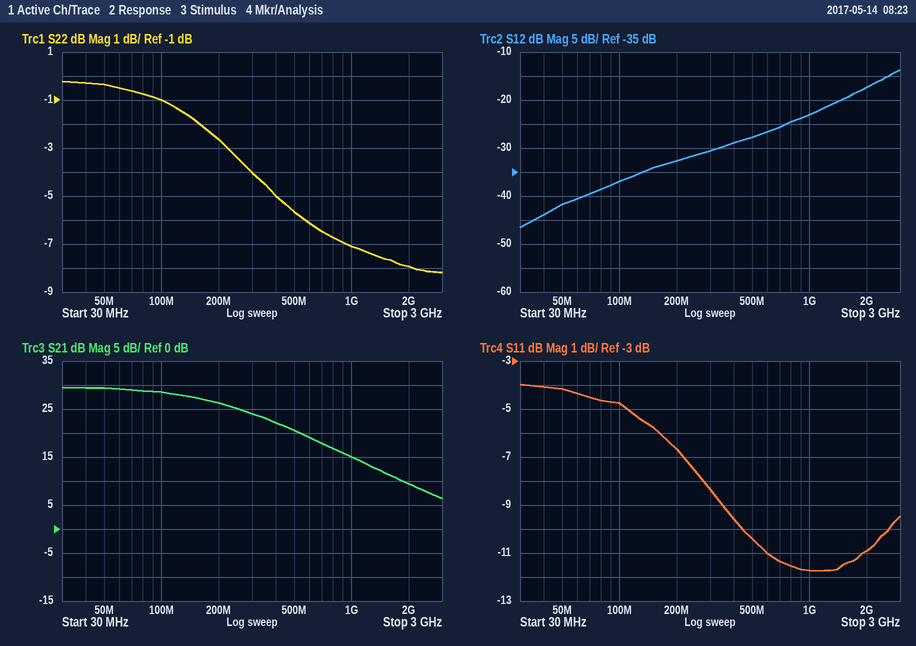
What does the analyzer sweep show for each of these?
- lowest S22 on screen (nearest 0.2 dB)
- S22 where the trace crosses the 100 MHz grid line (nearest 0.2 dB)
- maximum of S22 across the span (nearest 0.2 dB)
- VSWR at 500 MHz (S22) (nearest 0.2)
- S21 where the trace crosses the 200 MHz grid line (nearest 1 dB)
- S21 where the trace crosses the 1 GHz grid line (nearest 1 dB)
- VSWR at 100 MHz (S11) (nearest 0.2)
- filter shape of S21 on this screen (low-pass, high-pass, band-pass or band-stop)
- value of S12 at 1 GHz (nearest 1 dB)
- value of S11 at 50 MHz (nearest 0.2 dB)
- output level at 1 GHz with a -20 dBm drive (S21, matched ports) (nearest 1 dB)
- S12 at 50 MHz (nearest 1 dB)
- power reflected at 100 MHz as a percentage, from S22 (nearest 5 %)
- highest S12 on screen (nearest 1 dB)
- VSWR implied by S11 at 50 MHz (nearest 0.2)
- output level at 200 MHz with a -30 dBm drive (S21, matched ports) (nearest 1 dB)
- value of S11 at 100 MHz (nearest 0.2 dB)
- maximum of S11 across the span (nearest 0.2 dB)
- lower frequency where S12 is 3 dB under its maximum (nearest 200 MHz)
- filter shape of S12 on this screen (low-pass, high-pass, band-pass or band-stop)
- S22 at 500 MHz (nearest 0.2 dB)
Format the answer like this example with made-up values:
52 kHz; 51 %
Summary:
-8.2 dB; -1.0 dB; -0.2 dB; 3.2; 26 dB; 15 dB; 3.8; low-pass; -23 dB; -4.2 dB; -5 dBm; -42 dB; 80 %; -14 dB; 4.2; -4 dBm; -4.8 dB; -4.0 dB; 2.2 GHz; high-pass; -5.6 dB
